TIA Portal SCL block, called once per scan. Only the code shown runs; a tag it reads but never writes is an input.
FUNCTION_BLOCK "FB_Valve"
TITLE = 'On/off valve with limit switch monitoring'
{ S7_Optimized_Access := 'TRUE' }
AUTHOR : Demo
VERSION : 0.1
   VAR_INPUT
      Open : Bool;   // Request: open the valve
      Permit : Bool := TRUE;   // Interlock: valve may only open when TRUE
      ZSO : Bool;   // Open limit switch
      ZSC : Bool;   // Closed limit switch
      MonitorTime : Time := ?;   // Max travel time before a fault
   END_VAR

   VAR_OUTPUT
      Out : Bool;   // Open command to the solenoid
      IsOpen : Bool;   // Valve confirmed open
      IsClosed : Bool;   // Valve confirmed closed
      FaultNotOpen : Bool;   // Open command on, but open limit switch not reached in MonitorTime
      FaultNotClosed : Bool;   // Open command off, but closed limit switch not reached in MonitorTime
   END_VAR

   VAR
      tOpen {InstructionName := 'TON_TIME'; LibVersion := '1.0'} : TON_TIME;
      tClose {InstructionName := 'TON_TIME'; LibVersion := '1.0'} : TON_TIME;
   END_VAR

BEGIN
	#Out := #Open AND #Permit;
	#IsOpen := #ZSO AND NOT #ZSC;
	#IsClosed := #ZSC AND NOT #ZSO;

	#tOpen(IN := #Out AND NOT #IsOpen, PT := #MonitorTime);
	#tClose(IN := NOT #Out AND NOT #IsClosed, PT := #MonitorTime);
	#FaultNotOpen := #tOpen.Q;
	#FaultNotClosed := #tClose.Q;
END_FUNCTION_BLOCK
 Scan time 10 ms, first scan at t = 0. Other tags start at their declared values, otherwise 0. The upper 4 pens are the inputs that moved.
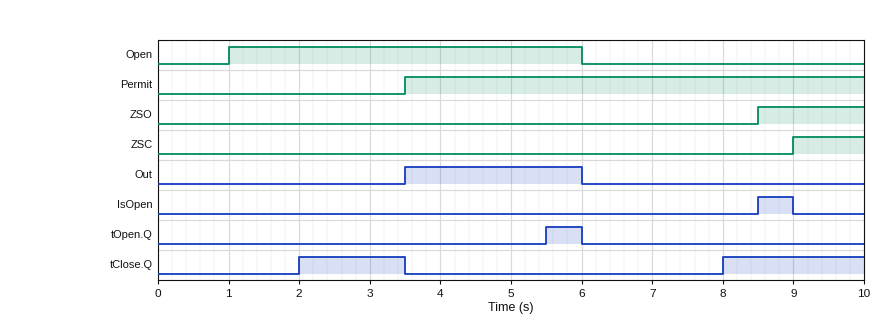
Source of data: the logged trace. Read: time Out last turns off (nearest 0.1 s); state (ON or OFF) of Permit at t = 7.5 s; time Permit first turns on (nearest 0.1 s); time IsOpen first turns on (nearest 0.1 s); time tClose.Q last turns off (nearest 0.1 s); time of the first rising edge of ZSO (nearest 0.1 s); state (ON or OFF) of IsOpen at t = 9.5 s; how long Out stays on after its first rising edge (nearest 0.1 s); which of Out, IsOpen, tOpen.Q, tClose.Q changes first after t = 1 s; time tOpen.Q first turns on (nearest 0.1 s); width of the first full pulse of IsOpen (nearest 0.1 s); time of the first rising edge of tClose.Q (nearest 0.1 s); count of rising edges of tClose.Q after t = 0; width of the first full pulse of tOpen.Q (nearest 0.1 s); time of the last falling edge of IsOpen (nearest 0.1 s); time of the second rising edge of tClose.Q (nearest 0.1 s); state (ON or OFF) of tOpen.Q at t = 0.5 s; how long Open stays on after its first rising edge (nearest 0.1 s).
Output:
6.0 s
ON
3.5 s
8.5 s
3.5 s
8.5 s
OFF
2.5 s
tClose.Q
5.5 s
0.5 s
2.0 s
2
0.5 s
9.0 s
8.0 s
OFF
5.0 s
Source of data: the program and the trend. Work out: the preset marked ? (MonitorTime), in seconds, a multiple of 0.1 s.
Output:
2.0 s
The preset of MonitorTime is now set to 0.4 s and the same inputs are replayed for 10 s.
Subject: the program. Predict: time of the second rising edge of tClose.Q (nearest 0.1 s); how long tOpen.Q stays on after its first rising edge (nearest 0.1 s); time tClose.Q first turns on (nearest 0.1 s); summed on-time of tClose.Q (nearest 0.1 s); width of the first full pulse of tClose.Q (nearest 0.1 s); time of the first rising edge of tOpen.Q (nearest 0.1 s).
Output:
6.4 s
2.1 s
0.4 s
6.7 s
3.1 s
3.9 s
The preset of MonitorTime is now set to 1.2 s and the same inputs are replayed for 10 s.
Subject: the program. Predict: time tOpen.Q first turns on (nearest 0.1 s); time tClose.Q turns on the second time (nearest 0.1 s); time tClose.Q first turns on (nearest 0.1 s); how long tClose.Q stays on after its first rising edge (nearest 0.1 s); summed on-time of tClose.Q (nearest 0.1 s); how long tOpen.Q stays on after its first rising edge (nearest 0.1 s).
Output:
4.7 s
7.2 s
1.2 s
2.3 s
5.1 s
1.3 s
